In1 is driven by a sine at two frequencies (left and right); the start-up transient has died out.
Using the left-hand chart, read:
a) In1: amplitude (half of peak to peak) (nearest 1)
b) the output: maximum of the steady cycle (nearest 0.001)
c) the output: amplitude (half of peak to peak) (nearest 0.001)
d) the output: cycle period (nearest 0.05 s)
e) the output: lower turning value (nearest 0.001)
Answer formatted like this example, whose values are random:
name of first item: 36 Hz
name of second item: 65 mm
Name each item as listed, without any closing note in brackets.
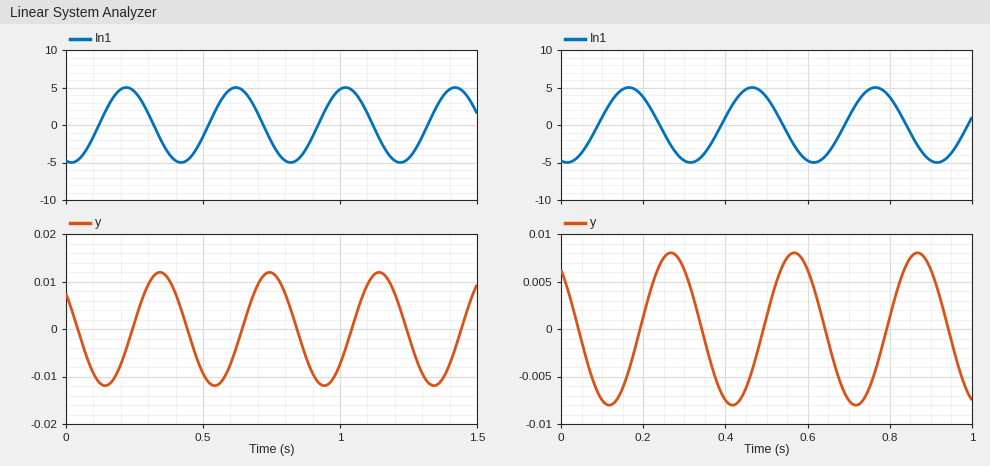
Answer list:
In1: amplitude (half of peak to peak): 5
the output: maximum of the steady cycle: 0.012
the output: amplitude (half of peak to peak): 0.012
the output: cycle period: 0.40 s
the output: lower turning value: -0.012
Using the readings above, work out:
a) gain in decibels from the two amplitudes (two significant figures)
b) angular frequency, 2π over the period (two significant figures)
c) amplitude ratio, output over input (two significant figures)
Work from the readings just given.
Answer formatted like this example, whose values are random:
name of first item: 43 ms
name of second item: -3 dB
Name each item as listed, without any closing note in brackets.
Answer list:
gain in decibels from the two amplitudes: -52 dB
angular frequency, 2π over the period: 16 rad/s
amplitude ratio, output over input: 0.0024
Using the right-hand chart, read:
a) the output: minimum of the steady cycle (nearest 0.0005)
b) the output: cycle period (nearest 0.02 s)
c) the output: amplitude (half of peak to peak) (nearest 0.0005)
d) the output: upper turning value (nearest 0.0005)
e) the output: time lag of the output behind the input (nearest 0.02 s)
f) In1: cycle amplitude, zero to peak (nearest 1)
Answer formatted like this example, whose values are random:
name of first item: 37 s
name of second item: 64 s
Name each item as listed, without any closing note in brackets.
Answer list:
the output: minimum of the steady cycle: -0.0080
the output: cycle period: 0.30 s
the output: amplitude (half of peak to peak): 0.0080
the output: upper turning value: 0.0080
the output: time lag of the output behind the input: 0.10 s
In1: cycle amplitude, zero to peak: 5
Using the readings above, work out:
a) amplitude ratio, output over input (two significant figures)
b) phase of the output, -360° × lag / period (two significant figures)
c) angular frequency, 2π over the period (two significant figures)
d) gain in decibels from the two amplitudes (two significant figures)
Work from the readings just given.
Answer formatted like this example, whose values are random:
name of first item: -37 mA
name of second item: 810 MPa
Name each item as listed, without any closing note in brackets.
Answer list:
amplitude ratio, output over input: 0.0016
phase of the output, -360° × lag / period: -120°
angular frequency, 2π over the period: 21 rad/s
gain in decibels from the two amplitudes: -56 dB
